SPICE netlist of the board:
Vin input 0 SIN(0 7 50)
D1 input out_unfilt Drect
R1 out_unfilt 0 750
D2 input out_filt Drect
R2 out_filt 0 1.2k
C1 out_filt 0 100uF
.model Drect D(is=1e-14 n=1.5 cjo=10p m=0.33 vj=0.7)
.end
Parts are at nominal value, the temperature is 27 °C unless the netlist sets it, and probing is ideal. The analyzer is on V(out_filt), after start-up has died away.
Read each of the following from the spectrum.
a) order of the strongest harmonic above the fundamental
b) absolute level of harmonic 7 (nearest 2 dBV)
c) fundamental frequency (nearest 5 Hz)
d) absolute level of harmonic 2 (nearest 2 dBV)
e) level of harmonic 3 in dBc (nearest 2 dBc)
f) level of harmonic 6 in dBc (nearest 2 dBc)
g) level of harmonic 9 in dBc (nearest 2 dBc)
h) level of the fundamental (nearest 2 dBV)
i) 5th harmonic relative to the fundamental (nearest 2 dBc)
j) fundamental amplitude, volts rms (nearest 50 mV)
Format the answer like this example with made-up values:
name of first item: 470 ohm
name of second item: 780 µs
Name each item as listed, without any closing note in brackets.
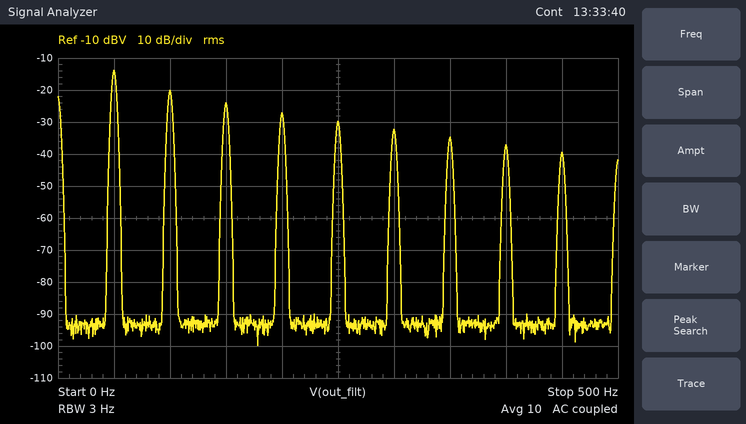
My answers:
order of the strongest harmonic above the fundamental: 2
absolute level of harmonic 7: -34 dBV
fundamental frequency: 50 Hz
absolute level of harmonic 2: -20 dBV
level of harmonic 3 in dBc: -10 dBc
level of harmonic 6 in dBc: -18 dBc
level of harmonic 9 in dBc: -26 dBc
level of the fundamental: -14 dBV
5th harmonic relative to the fundamental: -16 dBc
fundamental amplitude, volts rms: 200 mV
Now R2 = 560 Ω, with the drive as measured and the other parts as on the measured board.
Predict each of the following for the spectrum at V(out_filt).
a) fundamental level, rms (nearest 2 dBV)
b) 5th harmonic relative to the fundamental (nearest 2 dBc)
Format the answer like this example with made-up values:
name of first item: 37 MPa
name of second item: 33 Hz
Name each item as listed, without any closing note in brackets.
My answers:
fundamental level, rms: -8 dBV
5th harmonic relative to the fundamental: -18 dBc
